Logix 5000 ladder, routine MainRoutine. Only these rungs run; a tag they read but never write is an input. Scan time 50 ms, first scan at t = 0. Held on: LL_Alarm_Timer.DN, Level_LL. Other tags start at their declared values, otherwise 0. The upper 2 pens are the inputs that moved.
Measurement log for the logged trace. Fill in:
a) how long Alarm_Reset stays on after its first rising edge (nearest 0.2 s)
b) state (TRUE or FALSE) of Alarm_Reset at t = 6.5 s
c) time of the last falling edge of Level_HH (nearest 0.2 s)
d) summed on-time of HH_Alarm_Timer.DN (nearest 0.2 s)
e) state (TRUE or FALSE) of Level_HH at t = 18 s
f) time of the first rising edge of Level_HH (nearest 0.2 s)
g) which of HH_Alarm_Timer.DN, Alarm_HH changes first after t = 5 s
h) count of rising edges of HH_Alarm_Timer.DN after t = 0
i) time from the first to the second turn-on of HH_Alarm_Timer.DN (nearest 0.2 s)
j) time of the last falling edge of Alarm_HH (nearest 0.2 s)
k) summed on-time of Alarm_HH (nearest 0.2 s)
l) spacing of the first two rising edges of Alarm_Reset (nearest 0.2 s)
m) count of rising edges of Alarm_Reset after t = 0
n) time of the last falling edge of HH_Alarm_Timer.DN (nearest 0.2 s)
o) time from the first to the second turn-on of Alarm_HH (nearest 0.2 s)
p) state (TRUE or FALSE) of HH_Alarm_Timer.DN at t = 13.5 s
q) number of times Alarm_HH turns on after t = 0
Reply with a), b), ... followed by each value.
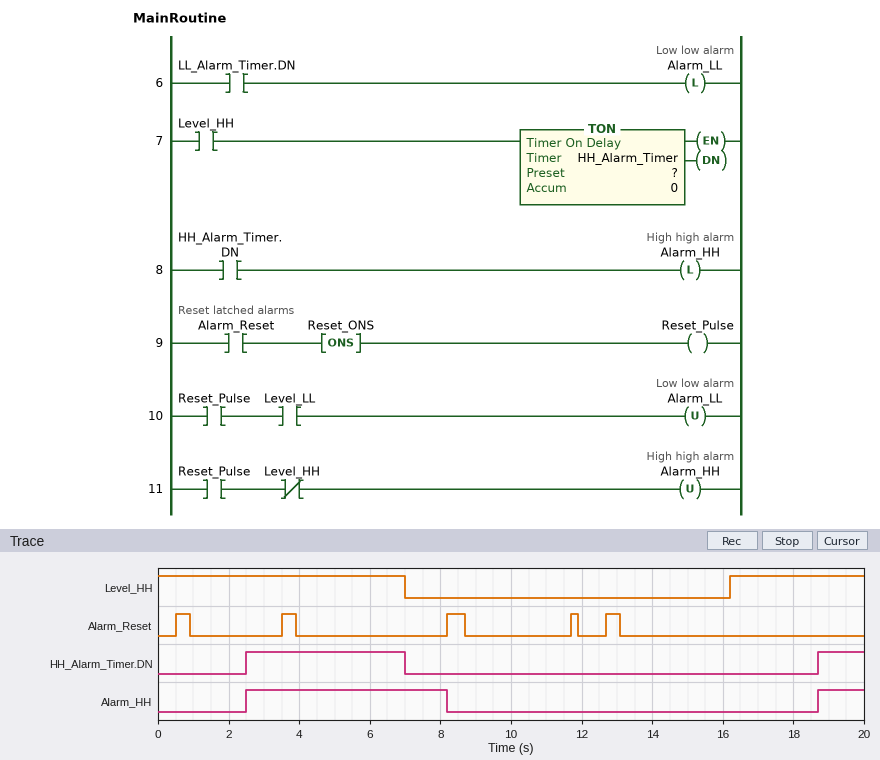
a) 0.4 s
b) FALSE
c) 7.0 s
d) 5.8 s
e) TRUE
f) 16.2 s
g) HH_Alarm_Timer.DN
h) 2
i) 16.2 s
j) 8.2 s
k) 7.0 s
l) 3.0 s
m) 5
n) 7.0 s
o) 16.2 s
p) FALSE
q) 2
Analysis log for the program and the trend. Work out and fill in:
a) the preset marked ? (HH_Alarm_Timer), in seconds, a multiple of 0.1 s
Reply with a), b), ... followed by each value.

a) 2.5 s
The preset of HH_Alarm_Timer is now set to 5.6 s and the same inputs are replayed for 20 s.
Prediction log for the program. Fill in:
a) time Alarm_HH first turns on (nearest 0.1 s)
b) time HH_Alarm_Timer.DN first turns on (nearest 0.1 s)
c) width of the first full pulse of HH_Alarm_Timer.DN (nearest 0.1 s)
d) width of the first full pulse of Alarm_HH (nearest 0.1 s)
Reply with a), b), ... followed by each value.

a) 5.6 s
b) 5.6 s
c) 1.4 s
d) 2.6 s
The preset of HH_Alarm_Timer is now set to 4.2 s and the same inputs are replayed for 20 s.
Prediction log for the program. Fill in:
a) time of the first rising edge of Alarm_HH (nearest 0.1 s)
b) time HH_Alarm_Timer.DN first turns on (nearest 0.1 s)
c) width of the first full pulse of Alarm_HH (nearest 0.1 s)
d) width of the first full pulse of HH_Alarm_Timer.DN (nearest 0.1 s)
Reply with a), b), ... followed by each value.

a) 4.2 s
b) 4.2 s
c) 4.0 s
d) 2.8 s
